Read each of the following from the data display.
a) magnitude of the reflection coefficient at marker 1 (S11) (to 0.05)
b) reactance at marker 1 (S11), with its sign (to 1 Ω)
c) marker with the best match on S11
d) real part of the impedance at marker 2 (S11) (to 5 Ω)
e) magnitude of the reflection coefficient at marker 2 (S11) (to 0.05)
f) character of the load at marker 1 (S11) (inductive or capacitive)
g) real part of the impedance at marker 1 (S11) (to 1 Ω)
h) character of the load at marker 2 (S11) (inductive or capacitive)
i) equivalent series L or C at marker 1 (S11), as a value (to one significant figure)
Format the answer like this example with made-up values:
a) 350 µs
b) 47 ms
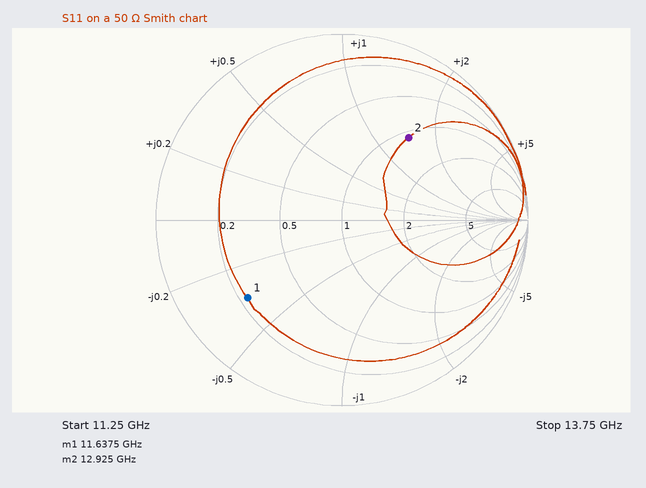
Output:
a) 0.65
b) -17 Ω
c) marker 2
d) 55 Ω
e) 0.55
f) capacitive
g) 12 Ω
h) inductive
i) 800 fF
